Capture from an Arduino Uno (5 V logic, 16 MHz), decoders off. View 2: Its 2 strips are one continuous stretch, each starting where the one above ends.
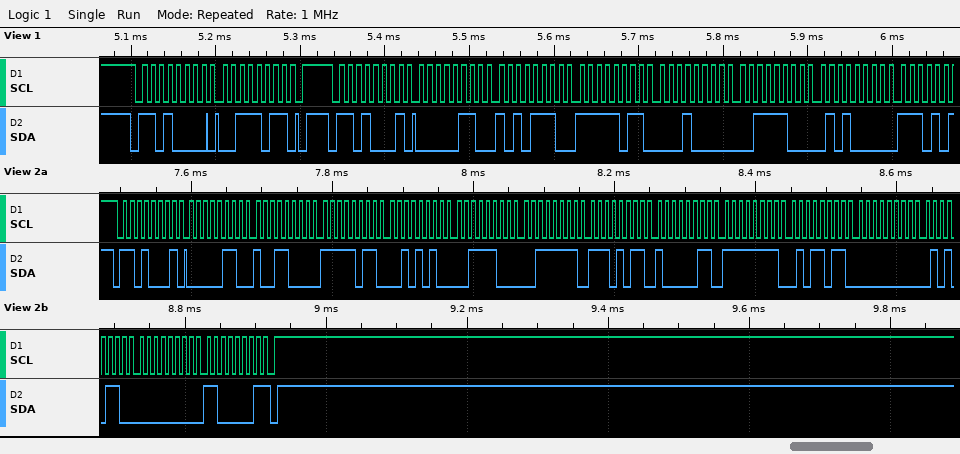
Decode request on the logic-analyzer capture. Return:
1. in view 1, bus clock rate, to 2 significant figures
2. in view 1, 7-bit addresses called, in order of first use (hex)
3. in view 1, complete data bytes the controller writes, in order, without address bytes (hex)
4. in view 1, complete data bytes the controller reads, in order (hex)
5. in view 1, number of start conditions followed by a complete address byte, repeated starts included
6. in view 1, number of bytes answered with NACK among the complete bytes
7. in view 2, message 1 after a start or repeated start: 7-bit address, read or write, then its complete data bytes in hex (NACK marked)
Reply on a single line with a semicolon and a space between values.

100 kHz; 0x68; 3B; 06 AE FB 10 3C 50; 2; 0; 0x68 read: 06 98 FB 2A 3C 3F EB 83 FF 5B 00 56 00 C1 NACK
